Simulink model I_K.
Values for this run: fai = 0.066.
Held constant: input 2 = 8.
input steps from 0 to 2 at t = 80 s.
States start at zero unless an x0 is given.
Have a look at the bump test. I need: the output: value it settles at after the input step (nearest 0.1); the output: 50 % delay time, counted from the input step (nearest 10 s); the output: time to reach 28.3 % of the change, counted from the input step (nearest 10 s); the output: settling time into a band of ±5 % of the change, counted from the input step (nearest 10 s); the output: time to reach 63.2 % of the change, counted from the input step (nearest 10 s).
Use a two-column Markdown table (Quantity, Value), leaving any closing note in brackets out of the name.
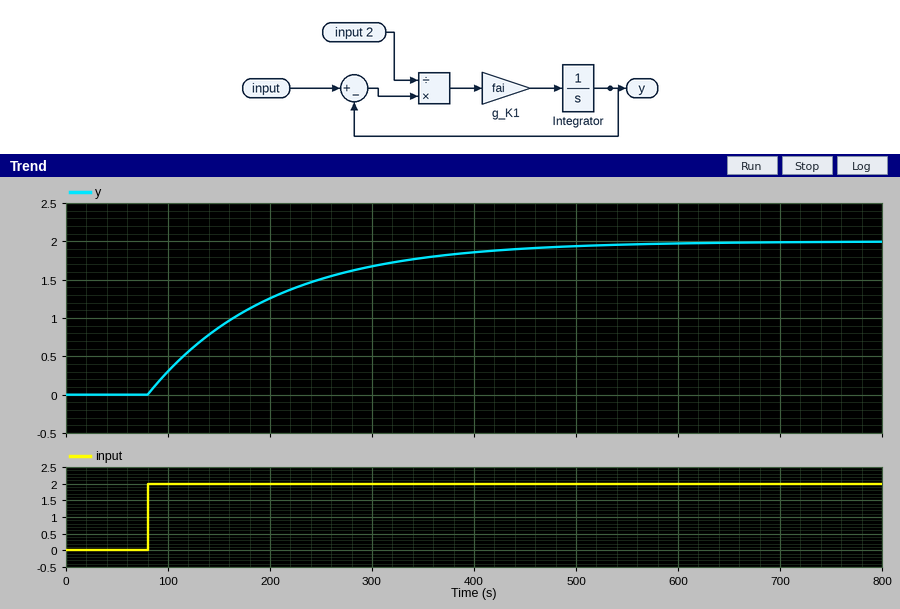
| Quantity | Value |
|---|---|
| the output: value it settles at after the input step | 2.0 |
| the output: 50 % delay time, counted from the input step | 80 s |
| the output: time to reach 28.3 % of the change, counted from the input step | 40 s |
| the output: settling time into a band of ±5 % of the change, counted from the input step | 360 s |
| the output: time to reach 63.2 % of the change, counted from the input step | 120 s |
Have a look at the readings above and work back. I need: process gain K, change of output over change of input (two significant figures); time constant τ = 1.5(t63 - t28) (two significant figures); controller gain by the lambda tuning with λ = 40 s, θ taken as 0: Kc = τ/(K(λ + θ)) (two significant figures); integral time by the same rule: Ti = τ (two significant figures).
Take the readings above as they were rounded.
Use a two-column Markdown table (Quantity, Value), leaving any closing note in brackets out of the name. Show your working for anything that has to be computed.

| Quantity | Value |
|---|---|
| process gain K, change of output over change of input | (2 - 0) / 2 = 1.0 |
| time constant τ = 1.5(t63 - t28) | 1.5 × (120 - 40) = 120 s |
| controller gain by the lambda tuning with λ = 40 s, θ taken as 0: Kc = τ/(K(λ + θ)) | 120 / (1 × (40 + 0)) = 3.0 |
| integral time by the same rule: Ti = τ | 120 s |
